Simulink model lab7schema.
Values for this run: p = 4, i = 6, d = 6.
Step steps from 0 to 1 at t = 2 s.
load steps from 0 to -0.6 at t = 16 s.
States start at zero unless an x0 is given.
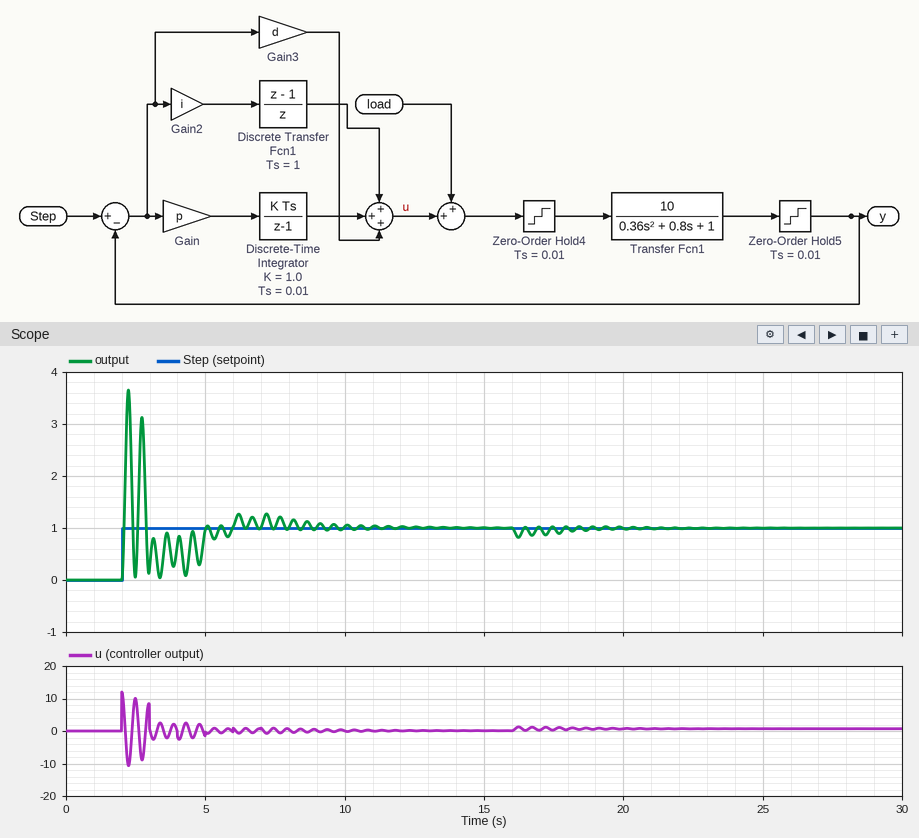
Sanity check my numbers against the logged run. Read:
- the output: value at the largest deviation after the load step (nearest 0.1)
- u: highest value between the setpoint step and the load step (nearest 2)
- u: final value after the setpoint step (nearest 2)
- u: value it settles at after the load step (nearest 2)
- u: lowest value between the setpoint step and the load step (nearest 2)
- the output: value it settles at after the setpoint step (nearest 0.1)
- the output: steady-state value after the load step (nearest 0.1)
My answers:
0.8
12
0
0
-10
1.0
1.0
